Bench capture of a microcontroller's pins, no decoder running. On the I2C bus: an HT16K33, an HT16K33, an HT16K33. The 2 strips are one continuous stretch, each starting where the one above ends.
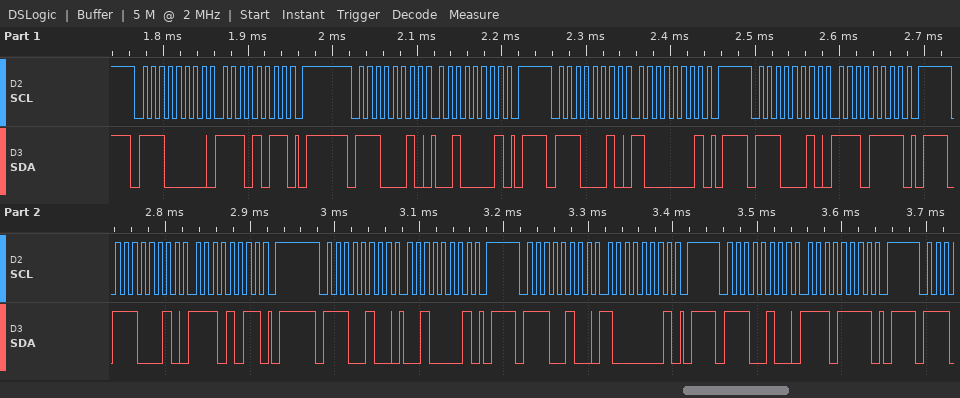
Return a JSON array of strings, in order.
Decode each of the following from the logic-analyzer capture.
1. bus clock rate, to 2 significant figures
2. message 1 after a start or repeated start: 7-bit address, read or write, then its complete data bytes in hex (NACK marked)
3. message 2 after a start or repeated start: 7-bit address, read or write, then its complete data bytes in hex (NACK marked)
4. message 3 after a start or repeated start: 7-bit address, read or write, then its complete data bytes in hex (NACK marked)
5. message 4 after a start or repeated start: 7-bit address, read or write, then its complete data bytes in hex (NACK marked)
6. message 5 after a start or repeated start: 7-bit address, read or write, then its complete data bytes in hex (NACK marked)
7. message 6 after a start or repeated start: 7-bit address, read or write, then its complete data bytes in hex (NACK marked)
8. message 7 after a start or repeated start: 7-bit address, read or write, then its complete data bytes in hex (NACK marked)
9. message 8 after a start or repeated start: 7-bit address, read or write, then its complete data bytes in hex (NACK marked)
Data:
["100 kHz", "0x70 write: EB", "0x71 write: 21", "0x71 write: 81", "0x71 write: EF", "0x71 write: EB", "0x72 write: 21", "0x72 write: 81", "0x72 write: EF"]
